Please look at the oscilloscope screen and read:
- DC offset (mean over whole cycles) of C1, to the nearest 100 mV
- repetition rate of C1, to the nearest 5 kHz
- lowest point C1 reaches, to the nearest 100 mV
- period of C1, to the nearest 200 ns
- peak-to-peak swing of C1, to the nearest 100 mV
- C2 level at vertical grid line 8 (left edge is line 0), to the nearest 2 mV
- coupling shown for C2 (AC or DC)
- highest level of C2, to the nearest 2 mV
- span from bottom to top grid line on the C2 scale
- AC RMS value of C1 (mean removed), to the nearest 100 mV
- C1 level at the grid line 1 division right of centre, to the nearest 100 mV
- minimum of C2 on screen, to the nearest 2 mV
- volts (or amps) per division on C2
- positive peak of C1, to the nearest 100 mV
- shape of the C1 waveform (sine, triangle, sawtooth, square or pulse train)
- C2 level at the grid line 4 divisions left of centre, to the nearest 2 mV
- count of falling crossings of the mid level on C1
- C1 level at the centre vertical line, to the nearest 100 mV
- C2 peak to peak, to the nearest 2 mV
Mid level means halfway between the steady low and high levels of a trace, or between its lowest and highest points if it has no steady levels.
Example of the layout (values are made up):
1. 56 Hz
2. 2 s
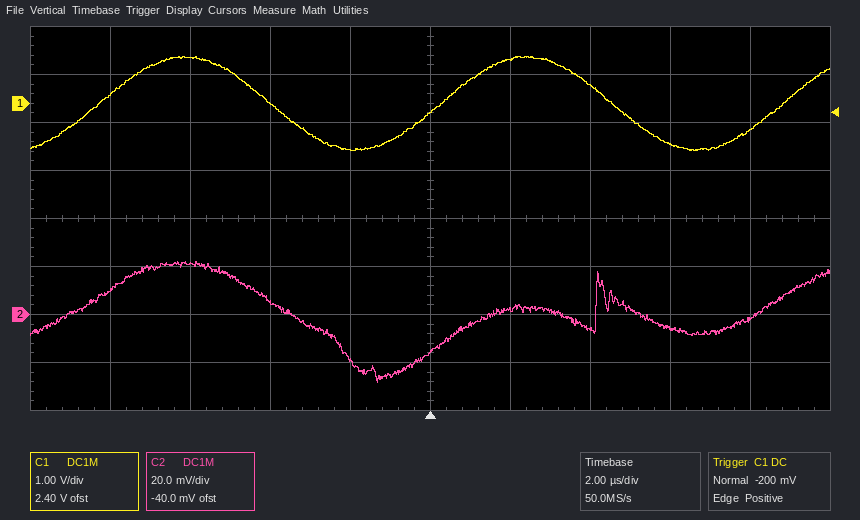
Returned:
1. 0.0 V
2. 115 kHz
3. -1.0 V
4. 8.6 µs
5. 2.0 V
6. -6 mV
7. DC
8. 22 mV
9. 160 mV
10. 700 mV
11. 900 mV
12. -28 mV
13. 20 mV
14. 1.0 V
15. sine
16. 10 mV
17. 2
18. -200 mV
19. 50 mV
